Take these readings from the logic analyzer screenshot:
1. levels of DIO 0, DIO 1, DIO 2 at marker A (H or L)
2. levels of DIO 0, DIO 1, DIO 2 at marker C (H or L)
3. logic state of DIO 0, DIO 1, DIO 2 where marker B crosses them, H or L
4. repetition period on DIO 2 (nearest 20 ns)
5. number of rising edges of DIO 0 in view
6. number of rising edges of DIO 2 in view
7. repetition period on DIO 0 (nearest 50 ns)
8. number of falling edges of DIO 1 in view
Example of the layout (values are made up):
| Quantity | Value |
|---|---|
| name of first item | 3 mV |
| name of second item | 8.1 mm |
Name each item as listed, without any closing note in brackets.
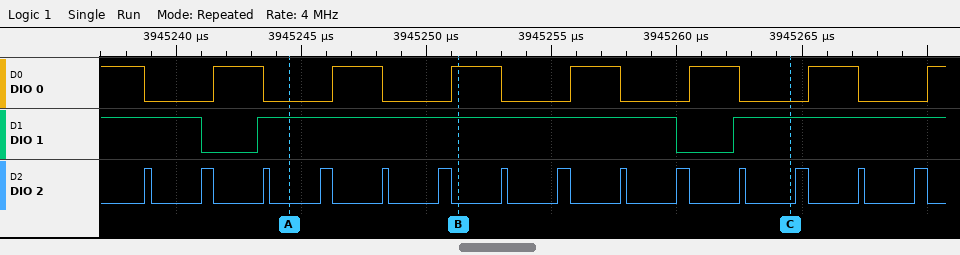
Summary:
| Quantity | Value |
|---|---|
| levels of DIO 0, DIO 1, DIO 2 at marker A | DIO 0=L, DIO 1=H, DIO 2=L |
| levels of DIO 0, DIO 1, DIO 2 at marker C | DIO 0=L, DIO 1=H, DIO 2=L |
| logic state of DIO 0, DIO 1, DIO 2 where marker B crosses them, H or L | DIO 0=H, DIO 1=H, DIO 2=L |
| repetition period on DIO 2 | 2360 ns |
| number of rising edges of DIO 0 in view | 7 |
| number of rising edges of DIO 2 in view | 14 |
| repetition period on DIO 0 | 4750 ns |
| number of falling edges of DIO 1 in view | 2 |
